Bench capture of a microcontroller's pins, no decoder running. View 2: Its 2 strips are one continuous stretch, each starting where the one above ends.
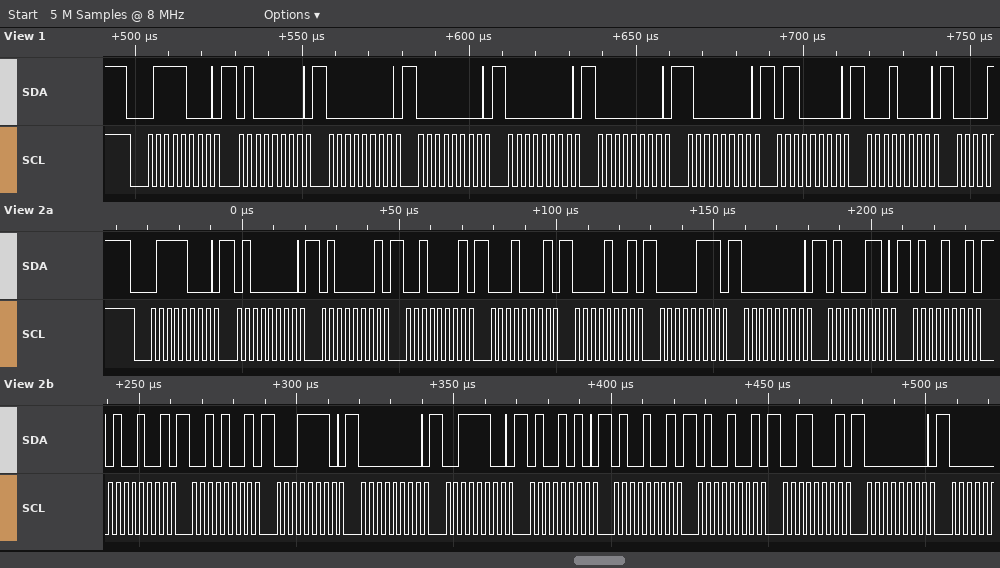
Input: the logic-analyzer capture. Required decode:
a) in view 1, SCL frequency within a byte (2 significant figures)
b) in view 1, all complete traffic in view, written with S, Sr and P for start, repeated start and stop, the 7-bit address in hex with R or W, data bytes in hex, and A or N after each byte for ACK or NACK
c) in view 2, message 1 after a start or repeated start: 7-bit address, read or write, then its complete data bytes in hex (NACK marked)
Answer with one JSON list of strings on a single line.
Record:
["400 kHz", "S 3CW A 40 A 00 A 00 A 00 A 00 A 80 A 60 A 10 A", "0x3C write: 40 41 21 11 09 07 00 46 49 49 29 1E 00 3C 4A 49 49 31 00"]
